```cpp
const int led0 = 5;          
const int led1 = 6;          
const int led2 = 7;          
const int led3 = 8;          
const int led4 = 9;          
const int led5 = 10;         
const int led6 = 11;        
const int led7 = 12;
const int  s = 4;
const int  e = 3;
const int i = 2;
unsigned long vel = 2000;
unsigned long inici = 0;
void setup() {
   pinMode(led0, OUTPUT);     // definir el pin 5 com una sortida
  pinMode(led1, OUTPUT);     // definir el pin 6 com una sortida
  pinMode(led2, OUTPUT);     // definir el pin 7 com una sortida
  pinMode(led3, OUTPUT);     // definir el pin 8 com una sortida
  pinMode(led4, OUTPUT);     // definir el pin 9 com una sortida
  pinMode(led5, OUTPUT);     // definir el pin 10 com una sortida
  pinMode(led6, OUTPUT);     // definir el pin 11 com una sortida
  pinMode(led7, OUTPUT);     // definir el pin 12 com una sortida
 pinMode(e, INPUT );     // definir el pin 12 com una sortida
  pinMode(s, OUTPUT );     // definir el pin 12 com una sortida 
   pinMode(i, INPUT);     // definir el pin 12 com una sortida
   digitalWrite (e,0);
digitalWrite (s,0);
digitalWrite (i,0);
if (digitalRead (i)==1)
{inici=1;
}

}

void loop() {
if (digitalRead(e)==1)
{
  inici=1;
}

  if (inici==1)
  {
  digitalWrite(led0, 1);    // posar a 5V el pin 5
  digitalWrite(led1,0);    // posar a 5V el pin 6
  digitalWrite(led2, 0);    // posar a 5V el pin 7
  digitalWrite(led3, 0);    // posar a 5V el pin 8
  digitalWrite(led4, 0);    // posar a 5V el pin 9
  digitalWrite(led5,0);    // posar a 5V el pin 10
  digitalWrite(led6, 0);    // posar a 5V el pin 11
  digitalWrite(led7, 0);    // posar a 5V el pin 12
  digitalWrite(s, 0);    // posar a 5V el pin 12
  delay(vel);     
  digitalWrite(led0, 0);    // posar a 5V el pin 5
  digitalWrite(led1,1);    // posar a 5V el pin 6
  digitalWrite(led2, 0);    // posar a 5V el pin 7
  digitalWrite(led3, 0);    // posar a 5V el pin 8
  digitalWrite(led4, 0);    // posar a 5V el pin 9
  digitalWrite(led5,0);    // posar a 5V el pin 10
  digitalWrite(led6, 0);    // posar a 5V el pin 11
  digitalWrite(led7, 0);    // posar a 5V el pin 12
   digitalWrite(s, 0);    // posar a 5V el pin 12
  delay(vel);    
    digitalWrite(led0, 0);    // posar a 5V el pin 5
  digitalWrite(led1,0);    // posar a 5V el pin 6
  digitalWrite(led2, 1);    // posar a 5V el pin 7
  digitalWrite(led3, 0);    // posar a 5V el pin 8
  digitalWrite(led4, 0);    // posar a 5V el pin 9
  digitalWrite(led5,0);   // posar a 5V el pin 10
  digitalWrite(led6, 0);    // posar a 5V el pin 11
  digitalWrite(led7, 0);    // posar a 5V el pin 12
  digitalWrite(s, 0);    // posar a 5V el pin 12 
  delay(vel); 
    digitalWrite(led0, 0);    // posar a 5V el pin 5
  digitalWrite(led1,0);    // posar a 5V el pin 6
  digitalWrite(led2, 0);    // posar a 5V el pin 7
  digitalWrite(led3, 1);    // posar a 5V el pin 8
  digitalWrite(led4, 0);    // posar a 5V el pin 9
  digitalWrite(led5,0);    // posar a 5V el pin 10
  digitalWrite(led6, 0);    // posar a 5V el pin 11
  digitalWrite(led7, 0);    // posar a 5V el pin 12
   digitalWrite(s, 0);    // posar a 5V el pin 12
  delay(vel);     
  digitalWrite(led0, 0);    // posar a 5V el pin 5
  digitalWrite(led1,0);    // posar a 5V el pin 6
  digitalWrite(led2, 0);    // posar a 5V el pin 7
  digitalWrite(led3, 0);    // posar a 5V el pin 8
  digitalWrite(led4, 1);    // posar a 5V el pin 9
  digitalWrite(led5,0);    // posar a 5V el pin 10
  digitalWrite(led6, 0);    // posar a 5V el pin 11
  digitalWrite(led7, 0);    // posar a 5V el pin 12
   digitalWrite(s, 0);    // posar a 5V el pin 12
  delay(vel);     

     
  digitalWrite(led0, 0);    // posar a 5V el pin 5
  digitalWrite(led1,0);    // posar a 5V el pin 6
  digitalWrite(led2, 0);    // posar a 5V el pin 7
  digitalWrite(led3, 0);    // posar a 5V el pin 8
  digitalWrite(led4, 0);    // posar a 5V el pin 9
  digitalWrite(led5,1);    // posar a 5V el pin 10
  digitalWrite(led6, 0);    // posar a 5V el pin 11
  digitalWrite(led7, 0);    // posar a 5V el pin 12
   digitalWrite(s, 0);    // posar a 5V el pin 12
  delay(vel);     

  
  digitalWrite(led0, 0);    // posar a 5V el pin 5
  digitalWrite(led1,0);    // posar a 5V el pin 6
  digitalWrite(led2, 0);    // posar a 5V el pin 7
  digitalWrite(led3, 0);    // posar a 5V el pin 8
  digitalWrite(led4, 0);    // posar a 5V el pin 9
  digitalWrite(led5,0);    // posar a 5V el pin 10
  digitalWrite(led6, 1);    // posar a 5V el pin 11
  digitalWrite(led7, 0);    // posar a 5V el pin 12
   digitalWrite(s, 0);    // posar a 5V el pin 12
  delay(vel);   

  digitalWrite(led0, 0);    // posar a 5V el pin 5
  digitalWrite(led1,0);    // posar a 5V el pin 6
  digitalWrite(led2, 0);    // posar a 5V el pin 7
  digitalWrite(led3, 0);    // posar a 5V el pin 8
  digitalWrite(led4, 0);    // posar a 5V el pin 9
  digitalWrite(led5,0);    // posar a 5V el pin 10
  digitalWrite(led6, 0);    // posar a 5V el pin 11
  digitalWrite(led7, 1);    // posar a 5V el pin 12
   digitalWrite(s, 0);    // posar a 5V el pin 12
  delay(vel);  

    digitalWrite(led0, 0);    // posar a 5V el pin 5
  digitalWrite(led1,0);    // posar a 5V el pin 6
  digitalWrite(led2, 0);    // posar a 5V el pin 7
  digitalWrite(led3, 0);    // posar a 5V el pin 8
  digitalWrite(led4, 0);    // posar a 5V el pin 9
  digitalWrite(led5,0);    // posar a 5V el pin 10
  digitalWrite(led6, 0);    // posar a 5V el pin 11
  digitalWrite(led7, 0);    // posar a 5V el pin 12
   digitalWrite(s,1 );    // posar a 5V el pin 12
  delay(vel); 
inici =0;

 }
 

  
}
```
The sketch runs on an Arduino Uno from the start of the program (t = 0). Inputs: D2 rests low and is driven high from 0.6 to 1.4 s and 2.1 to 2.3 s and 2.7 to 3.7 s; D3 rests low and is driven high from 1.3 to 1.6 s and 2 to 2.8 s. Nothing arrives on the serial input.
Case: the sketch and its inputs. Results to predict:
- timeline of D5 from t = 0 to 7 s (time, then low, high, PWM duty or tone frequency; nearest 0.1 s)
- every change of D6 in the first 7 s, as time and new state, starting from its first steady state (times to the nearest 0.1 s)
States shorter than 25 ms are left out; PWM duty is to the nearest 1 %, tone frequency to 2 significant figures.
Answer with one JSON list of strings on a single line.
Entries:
["0 s low; 1.3 s high; 3.3 s low", "0 s low; 3.3 s high; 5.3 s low"]
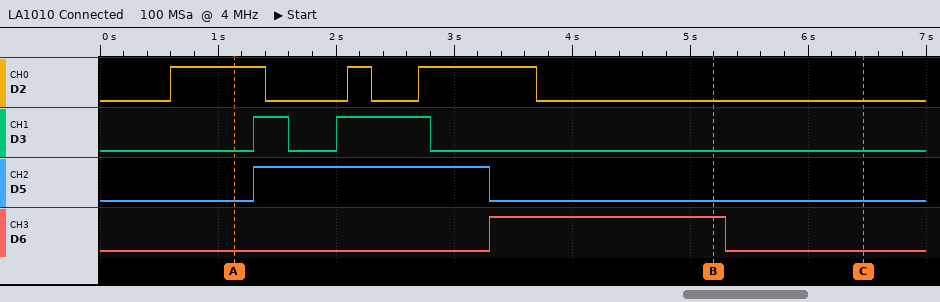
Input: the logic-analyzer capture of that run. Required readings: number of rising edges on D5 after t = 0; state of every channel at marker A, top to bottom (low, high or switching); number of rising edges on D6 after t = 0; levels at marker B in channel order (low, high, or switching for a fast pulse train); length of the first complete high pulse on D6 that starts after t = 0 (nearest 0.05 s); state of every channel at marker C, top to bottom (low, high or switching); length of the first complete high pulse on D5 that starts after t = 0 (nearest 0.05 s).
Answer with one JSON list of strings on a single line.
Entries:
["1", "D2 high, D3 low, D5 low, D6 low", "1", "D2 low, D3 low, D5 low, D6 high", "2.00 s", "D2 low, D3 low, D5 low, D6 low", "2.00 s"]
